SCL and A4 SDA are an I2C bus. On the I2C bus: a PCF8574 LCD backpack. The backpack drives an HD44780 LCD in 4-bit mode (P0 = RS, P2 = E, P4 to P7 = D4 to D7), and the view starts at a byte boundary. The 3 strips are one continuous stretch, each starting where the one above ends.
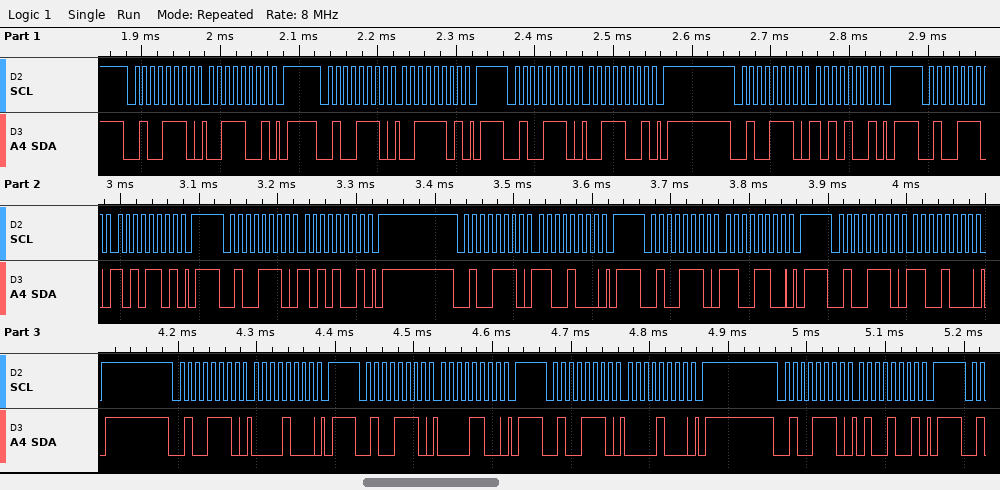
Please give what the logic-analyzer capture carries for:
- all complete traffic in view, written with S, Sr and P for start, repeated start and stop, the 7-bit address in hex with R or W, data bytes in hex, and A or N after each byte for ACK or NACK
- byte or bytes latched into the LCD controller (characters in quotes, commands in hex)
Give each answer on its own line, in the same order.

S 27W A 39 A P S 27W A 3D A P S 27W A 39 A P S 27W A A9 A P S 27W A AD A P S 27W A A9 A P S 27W A C8 A P S 27W A CC A P S 27W A C8 A P S 27W A 08 A P S 27W A 0C A P S 27W A 08 A P S 27W A 49 A P
':' 0xC0
